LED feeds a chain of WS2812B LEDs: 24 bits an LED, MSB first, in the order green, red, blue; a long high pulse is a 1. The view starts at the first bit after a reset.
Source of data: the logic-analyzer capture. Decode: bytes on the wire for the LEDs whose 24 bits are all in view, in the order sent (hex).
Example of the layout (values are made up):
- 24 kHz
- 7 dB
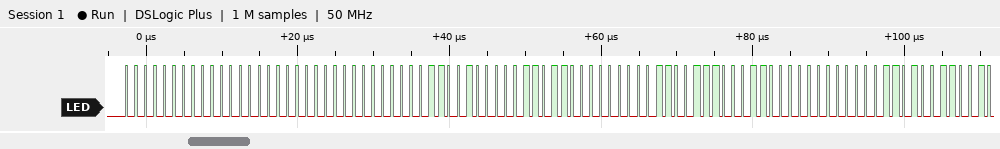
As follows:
- 00 00 00 00 C8 36 00 CE 30
